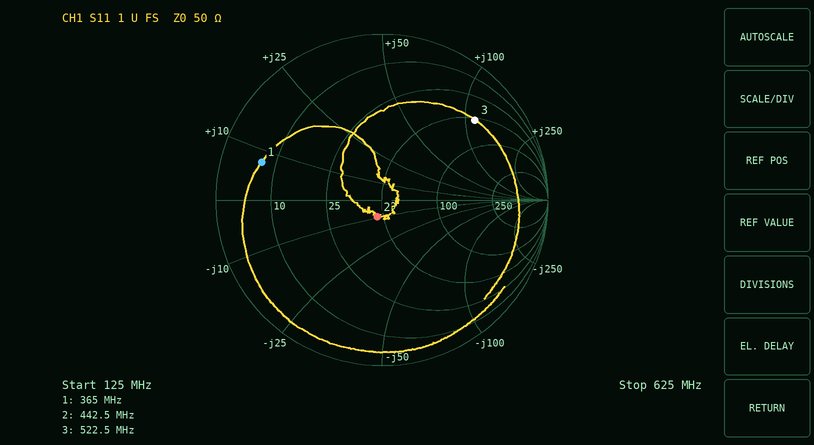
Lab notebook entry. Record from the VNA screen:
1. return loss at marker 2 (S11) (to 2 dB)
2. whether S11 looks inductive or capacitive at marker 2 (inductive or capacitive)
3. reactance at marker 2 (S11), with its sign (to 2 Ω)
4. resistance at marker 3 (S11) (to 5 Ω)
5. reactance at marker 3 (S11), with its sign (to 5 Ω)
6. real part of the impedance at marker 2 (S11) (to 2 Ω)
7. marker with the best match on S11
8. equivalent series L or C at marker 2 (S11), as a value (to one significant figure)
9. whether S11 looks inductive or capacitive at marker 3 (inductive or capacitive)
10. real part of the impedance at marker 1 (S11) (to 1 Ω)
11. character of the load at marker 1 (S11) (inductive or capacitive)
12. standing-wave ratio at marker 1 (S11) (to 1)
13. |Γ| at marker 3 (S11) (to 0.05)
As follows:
20 dB
capacitive
-10 Ω
55 Ω
+115 Ω
46 Ω
marker 2
40 pF
inductive
7 Ω
inductive
7
0.75
